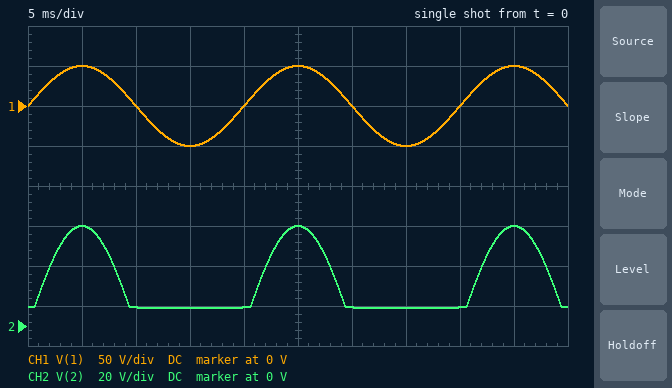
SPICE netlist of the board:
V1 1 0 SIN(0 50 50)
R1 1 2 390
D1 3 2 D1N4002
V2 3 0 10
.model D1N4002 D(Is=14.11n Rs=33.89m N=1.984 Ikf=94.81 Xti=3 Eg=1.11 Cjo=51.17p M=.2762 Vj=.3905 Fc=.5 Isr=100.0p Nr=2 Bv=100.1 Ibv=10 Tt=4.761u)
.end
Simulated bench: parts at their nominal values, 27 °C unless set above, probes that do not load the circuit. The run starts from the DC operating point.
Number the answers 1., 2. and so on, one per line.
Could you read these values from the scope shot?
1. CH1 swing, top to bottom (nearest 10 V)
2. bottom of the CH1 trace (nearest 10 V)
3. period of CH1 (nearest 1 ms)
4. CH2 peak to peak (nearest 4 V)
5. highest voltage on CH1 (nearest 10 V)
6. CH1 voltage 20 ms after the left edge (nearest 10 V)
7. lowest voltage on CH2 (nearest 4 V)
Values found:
1. 100 V
2. -50 V
3. 20 ms
4. 40 V
5. 50 V
6. 0 V
7. 8 V
